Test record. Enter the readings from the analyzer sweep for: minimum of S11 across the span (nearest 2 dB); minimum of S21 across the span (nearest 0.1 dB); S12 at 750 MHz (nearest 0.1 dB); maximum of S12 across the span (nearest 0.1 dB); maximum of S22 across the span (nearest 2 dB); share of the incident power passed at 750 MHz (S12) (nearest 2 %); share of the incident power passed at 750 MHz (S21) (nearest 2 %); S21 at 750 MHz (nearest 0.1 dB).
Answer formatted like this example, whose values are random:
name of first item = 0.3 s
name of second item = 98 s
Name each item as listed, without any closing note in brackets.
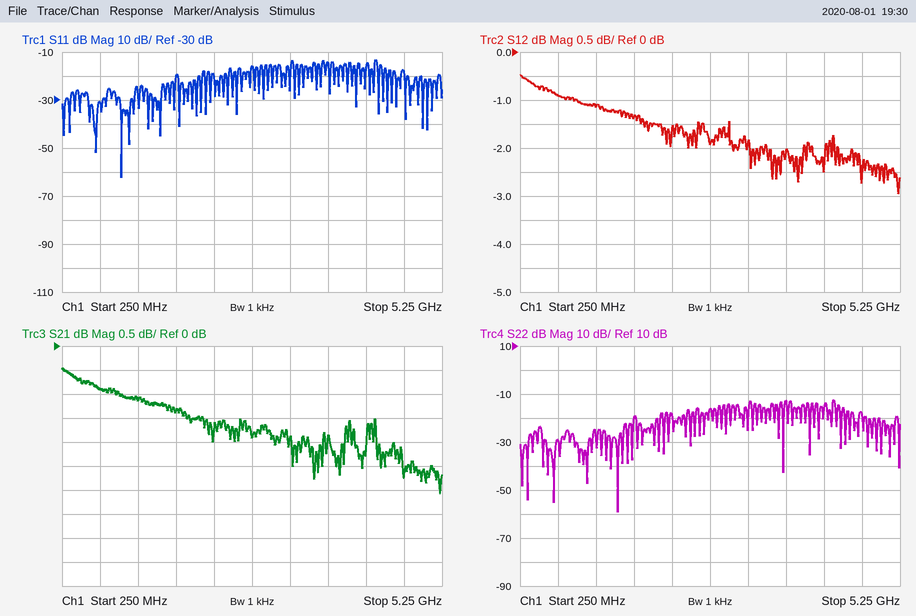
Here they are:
minimum of S11 across the span = -62 dB
minimum of S21 across the span = -3.1 dB
S12 at 750 MHz = -0.9 dB
maximum of S12 across the span = -0.5 dB
maximum of S22 across the span = -12 dB
share of the incident power passed at 750 MHz (S12) = 82 %
share of the incident power passed at 750 MHz (S21) = 82 %
S21 at 750 MHz = -0.9 dB
